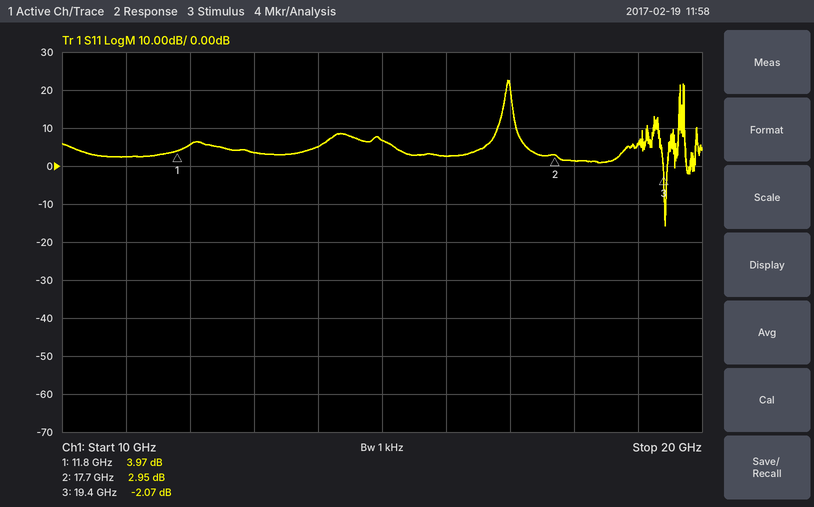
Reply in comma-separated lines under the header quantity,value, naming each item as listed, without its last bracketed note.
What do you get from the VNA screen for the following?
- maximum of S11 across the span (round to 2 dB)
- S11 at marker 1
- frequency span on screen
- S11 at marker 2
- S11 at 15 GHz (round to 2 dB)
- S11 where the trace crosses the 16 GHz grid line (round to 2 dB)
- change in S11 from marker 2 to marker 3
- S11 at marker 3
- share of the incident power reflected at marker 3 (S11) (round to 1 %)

quantity,value
maximum of S11 across the span,22 dB
S11 at marker 1,3.97 dB
frequency span on screen,10 GHz
S11 at marker 2,2.95 dB
S11 at 15 GHz,6 dB
S11 where the trace crosses the 16 GHz grid line,2 dB
change in S11 from marker 2 to marker 3,-5.02 dB
S11 at marker 3,-2.07 dB
share of the incident power reflected at marker 3 (S11),62 %
